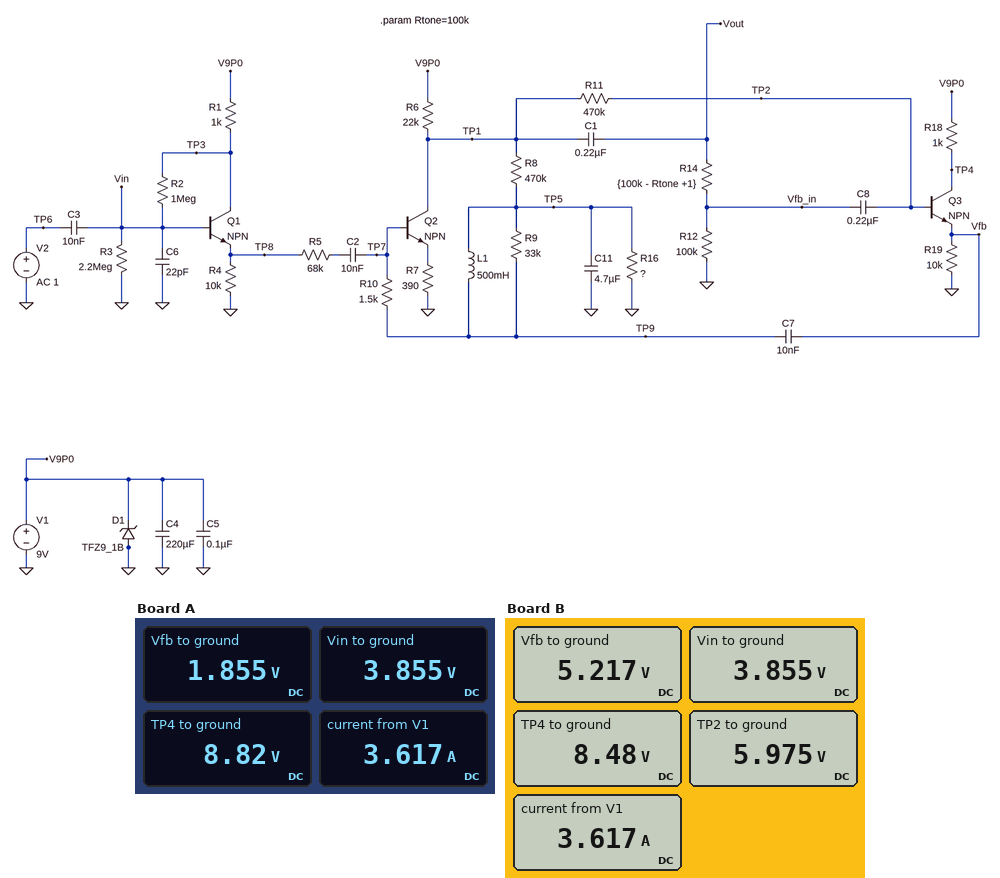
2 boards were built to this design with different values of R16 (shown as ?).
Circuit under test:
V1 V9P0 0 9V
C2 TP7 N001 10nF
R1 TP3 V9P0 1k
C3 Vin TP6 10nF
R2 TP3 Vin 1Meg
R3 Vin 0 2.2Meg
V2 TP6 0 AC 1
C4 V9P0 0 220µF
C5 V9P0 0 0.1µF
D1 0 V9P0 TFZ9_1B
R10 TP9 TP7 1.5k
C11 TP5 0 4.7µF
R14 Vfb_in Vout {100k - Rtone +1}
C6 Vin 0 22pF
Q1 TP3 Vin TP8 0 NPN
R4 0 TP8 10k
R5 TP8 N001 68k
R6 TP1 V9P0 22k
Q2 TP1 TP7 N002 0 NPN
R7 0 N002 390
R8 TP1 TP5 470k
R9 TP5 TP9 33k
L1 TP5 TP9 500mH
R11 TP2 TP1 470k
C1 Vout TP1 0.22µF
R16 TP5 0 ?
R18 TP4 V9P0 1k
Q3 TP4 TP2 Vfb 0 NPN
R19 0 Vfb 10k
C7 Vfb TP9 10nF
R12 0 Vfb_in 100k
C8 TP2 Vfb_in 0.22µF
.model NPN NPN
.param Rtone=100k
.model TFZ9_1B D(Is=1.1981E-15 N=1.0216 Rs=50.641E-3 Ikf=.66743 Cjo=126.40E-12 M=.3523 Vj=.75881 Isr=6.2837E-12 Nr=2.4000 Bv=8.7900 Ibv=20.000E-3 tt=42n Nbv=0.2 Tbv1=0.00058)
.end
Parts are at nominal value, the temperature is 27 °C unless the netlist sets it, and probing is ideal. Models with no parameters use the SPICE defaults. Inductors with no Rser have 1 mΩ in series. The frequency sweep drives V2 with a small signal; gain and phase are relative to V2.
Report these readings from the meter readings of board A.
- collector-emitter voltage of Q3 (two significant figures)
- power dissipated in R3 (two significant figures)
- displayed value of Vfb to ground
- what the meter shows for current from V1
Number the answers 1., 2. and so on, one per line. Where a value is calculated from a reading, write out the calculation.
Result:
1. 8.82 V - 1.855 V = 7.0 V
2. (3.855 V)^2 / 2.2 MΩ = 6.8 µW
3. 1.855 V
4. 3.617 A
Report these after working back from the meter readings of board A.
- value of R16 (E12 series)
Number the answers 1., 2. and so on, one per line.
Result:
1. 270 kΩ
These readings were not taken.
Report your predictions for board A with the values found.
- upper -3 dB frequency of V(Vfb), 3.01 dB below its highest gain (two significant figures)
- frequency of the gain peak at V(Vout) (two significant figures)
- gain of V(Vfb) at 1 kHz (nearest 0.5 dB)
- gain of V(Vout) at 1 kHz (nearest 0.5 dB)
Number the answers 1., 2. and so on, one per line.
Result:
1. 420 Hz
2. 400 Hz
3. -11.0 dB
4. -10.5 dB
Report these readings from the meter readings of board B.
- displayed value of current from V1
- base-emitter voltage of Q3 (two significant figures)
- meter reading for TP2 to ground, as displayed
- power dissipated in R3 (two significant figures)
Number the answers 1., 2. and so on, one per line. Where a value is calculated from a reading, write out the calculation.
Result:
1. 3.617 A
2. 5.975 V - 5.217 V = 760 mV
3. 5.975 V
4. (3.855 V)^2 / 2.2 MΩ = 6.8 µW
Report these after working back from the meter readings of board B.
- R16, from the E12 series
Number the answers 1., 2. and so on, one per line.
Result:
1. 39 kΩ
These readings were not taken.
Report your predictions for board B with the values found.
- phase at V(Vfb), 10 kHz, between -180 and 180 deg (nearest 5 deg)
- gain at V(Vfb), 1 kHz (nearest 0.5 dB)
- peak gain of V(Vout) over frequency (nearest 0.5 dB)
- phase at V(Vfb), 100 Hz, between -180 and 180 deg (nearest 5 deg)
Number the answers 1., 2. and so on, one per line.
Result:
1. 130 deg
2. -3.0 dB
3. 0 dB
4. -90 deg
